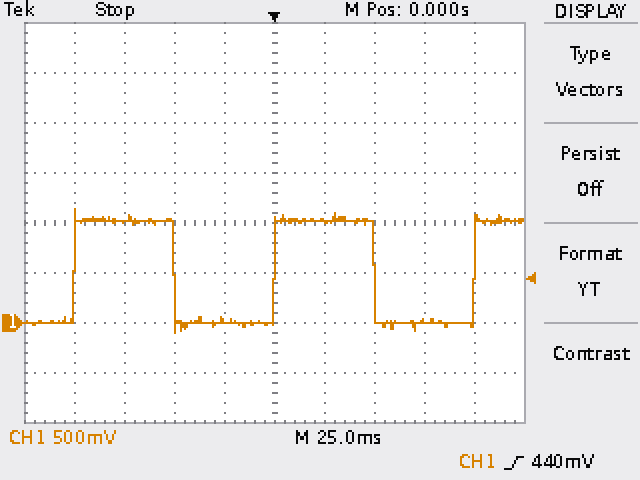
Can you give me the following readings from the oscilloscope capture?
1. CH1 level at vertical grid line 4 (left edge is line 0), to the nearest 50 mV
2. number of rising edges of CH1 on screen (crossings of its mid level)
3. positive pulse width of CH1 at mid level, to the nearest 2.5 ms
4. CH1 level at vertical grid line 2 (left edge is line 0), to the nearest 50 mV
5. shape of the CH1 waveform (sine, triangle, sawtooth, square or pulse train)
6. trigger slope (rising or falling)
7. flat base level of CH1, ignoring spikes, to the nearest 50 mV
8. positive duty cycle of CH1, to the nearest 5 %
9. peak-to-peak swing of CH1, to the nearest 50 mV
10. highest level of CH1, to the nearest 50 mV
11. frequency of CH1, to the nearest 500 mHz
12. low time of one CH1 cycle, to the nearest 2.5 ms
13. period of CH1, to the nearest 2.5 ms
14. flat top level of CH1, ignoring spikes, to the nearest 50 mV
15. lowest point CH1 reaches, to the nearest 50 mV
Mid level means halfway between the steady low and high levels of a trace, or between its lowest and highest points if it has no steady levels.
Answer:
50 mV
3
50.0 ms
1.00 V
square
rising
0 mV
50 %
1.25 V
1.15 V
10.0 Hz
50.0 ms
100.0 ms
1.00 V
-100 mV
